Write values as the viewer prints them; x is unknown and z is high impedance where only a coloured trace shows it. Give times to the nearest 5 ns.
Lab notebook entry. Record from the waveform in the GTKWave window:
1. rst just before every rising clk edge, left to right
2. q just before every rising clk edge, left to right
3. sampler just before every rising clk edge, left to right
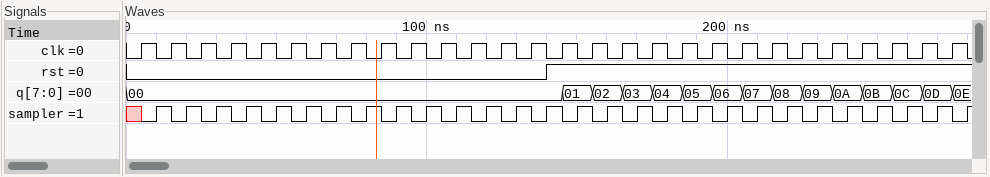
0 0 0 0 0 0 0 0 0 0 0 0 0 0 1 1 1 1 1 1 1 1 1 1 1 1 1 1
00, 00, 00, 00, 00, 00, 00, 00, 00, 00, 00, 00, 00, 00, 00, 01, 02, 03, 04, 05, 06, 07, 08, 09, 0A, 0B, 0C, 0D
x 1 1 1 1 1 1 1 1 1 1 1 1 1 1 1 1 1 1 1 1 1 1 1 1 1 1 1
